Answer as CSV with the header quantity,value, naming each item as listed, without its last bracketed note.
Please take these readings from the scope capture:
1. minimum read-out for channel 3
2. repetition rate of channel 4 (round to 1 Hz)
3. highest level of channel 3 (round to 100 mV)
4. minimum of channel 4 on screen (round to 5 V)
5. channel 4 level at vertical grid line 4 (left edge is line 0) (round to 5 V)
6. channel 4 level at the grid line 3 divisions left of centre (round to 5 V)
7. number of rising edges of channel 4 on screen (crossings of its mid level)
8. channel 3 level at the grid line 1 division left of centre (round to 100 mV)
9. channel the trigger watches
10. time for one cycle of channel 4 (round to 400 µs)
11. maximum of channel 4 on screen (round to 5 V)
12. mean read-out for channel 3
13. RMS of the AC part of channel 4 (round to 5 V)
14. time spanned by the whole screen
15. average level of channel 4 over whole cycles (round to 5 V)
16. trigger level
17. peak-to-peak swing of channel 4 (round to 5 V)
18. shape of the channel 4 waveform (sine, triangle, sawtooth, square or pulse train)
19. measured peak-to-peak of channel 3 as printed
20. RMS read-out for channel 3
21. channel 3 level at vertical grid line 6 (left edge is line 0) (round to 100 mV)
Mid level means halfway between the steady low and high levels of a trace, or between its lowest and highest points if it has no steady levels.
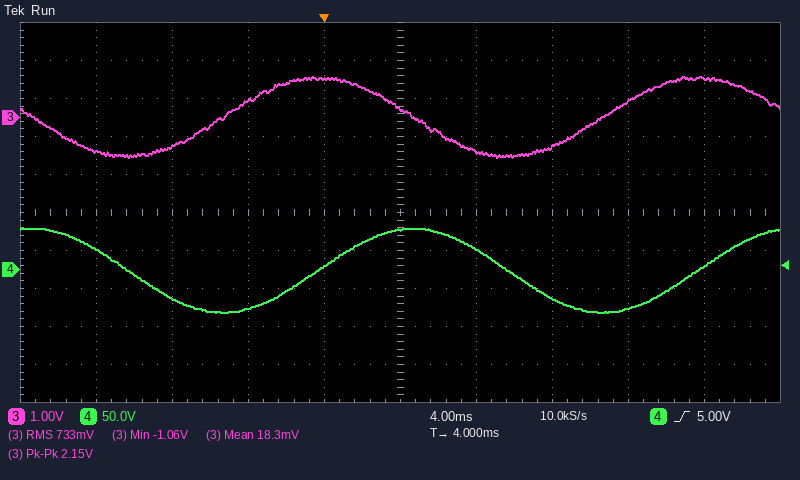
quantity,value
minimum read-out for channel 3,-1.06 V
repetition rate of channel 4,50 Hz
highest level of channel 3,1.1 V
minimum of channel 4 on screen,-55 V
channel 4 level at vertical grid line 4 (left edge is line 0),5 V
channel 4 level at the grid line 3 divisions left of centre,-40 V
number of rising edges of channel 4 on screen,2
channel 3 level at the grid line 1 division left of centre,1.0 V
channel the trigger watches,channel 4
time for one cycle of channel 4,20.0 ms
maximum of channel 4 on screen,55 V
mean read-out for channel 3,18.3 mV
RMS of the AC part of channel 4,40 V
time spanned by the whole screen,40 ms
average level of channel 4 over whole cycles,0 V
trigger level,5.00 V
peak-to-peak swing of channel 4,110 V
shape of the channel 4 waveform,sine
measured peak-to-peak of channel 3 as printed,2.15 V
RMS read-out for channel 3,733 mV
channel 3 level at vertical grid line 6 (left edge is line 0),-900 mV
